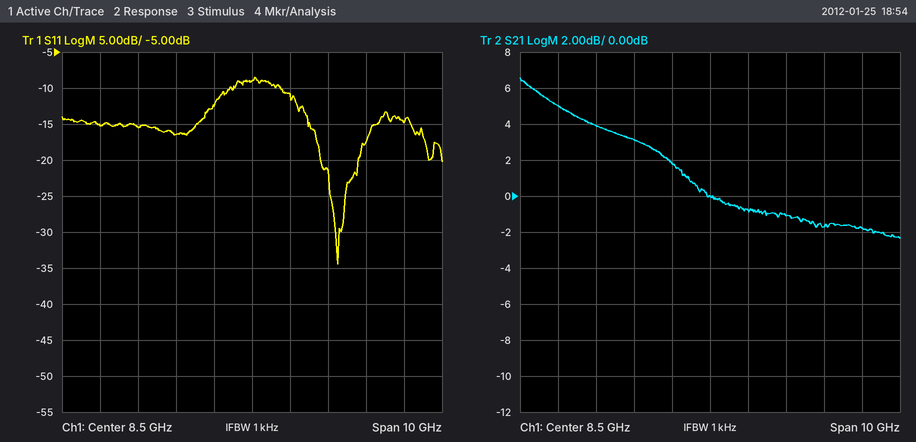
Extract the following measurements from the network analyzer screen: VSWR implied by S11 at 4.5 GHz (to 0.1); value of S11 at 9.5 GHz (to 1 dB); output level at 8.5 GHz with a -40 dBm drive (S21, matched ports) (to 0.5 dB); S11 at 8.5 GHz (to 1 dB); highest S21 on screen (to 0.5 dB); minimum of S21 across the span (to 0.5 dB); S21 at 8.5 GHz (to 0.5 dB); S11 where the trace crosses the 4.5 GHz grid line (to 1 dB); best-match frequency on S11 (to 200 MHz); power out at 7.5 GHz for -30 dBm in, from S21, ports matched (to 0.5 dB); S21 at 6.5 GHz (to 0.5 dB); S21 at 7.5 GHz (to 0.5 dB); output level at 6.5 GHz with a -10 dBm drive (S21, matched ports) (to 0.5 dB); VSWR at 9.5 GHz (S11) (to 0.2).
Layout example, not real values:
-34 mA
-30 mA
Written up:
1.4
-11 dB
-40.0 dBm
-9 dB
6.5 dB
-2.5 dB
0.0 dB
-15 dB
10.8 GHz
-28.0 dBm
3.0 dB
2.0 dB
-7.0 dBm
1.8
